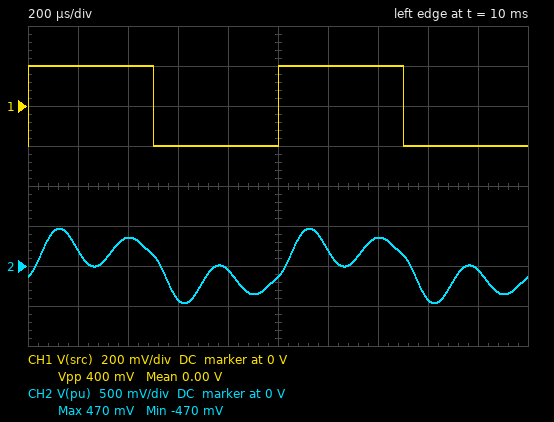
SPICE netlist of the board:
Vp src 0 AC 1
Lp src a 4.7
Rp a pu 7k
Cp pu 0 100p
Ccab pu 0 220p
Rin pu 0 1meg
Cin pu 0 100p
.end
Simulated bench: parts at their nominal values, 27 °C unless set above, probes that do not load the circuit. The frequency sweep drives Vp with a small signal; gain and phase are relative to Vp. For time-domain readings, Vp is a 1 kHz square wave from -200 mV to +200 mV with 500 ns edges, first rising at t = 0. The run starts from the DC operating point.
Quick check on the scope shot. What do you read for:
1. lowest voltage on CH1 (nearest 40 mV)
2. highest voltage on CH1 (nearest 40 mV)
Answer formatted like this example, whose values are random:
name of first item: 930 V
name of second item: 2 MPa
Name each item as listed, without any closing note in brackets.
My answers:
lowest voltage on CH1: -200 mV
highest voltage on CH1: 200 mV
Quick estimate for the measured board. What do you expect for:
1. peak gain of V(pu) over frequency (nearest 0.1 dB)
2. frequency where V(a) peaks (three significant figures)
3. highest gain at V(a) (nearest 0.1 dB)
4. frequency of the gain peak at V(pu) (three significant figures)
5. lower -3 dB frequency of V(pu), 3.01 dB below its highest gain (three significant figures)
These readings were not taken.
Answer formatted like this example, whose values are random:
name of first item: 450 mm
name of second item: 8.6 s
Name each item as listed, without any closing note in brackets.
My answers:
peak gain of V(pu) over frequency: 15.3 dB
frequency where V(a) peaks: 3.57 kHz
highest gain at V(a): 15.4 dB
frequency of the gain peak at V(pu): 3.57 kHz
lower -3 dB frequency of V(pu), 3.01 dB below its highest gain: 3.24 kHz
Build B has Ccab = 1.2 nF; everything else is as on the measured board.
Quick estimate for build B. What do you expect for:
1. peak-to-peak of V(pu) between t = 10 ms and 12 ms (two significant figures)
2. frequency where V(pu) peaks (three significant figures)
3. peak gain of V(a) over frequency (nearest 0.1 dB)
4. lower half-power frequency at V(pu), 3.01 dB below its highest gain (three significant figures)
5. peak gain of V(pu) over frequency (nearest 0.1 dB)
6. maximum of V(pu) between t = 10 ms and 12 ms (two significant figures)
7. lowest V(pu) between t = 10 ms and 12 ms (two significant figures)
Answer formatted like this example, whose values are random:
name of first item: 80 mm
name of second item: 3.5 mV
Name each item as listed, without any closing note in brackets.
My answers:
peak-to-peak of V(pu) between t = 10 ms and 12 ms: 780 mV
frequency where V(pu) peaks: 1.95 kHz
peak gain of V(a) over frequency: 15.1 dB
lower half-power frequency at V(pu), 3.01 dB below its highest gain: 1.77 kHz
peak gain of V(pu) over frequency: 15.0 dB
maximum of V(pu) between t = 10 ms and 12 ms: 390 mV
lowest V(pu) between t = 10 ms and 12 ms: -390 mV
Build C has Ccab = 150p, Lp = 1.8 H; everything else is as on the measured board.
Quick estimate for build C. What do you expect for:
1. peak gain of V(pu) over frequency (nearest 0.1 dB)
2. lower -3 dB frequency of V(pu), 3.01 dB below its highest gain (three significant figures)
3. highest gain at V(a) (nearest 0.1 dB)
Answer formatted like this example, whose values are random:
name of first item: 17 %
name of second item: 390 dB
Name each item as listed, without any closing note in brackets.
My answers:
peak gain of V(pu) over frequency: 15.4 dB
lower -3 dB frequency of V(pu), 3.01 dB below its highest gain: 5.75 kHz
highest gain at V(a): 15.5 dB
